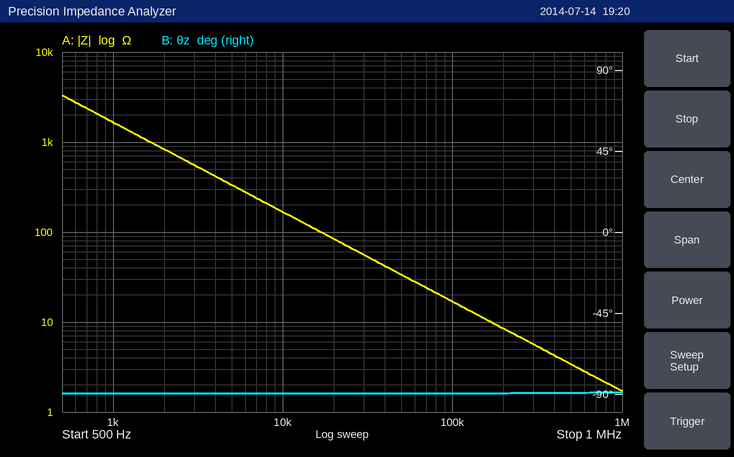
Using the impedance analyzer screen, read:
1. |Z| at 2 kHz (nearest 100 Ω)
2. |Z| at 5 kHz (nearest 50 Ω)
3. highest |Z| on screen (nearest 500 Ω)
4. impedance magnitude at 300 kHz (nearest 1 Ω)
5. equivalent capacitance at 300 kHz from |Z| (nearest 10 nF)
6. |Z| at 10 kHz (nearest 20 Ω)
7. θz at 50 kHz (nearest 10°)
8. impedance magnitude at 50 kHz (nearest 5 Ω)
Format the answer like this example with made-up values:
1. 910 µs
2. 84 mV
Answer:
1. 800 Ω
2. 350 Ω
3. 3.5 kΩ
4. 6 Ω
5. 90 nF
6. 160 Ω
7. -90°
8. 35 Ω
